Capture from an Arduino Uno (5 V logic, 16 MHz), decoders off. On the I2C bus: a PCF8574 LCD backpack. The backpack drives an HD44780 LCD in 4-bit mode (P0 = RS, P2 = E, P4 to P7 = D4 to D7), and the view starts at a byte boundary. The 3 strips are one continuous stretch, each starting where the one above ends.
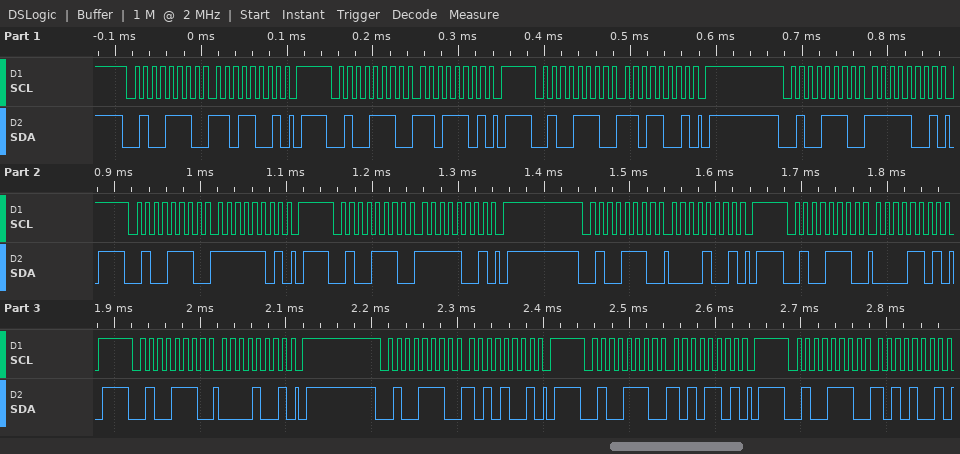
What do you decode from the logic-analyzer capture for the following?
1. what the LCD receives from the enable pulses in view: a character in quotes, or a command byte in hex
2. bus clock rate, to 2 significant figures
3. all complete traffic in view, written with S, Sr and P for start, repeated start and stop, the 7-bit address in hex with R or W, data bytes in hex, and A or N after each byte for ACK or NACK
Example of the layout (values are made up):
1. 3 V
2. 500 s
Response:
1. data 0xDF data 0x0A
2. 100 kHz
3. S 27W A D9 A P S 27W A DD A P S 27W A D9 A P S 27W A F9 A P S 27W A FD A P S 27W A F9 A P S 27W A 09 A P S 27W A 0D A P S 27W A 09 A P S 27W A A9 A P S 27W A AD A P S 27W A A9 A
